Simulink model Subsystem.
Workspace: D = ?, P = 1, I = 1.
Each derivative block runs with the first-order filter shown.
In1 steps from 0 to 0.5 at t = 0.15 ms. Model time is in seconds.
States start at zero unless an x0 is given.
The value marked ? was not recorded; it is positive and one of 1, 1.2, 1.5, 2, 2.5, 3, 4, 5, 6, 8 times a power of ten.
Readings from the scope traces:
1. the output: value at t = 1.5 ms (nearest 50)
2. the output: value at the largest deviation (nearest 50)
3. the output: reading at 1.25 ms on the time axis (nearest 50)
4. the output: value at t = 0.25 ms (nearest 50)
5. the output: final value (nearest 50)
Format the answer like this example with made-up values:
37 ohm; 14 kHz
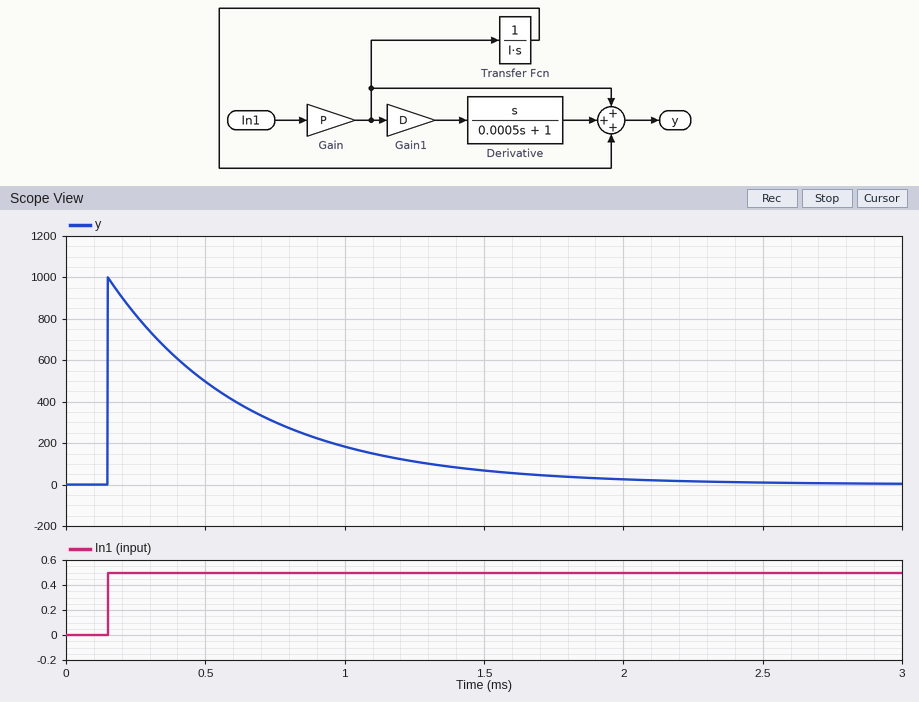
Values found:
50; 1000; 100; 800; 0
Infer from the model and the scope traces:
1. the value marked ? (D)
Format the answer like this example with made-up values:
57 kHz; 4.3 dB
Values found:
1
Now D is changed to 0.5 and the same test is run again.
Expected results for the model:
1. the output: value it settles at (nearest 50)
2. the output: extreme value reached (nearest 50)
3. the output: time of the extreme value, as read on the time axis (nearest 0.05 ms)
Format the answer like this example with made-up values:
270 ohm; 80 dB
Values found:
0; 500; 0.15 ms
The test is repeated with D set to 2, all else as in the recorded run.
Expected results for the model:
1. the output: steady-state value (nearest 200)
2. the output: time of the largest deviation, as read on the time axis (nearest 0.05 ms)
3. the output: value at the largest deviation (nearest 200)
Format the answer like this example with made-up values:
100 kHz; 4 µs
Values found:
0; 0.15 ms; 2000
